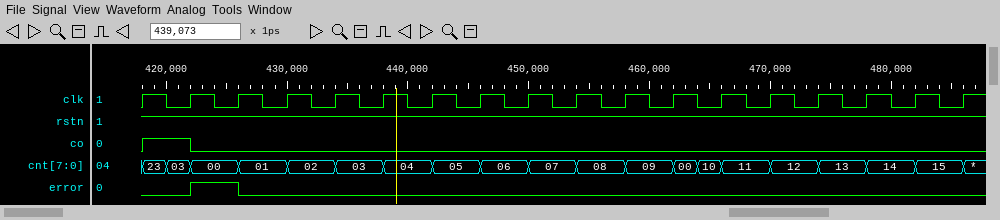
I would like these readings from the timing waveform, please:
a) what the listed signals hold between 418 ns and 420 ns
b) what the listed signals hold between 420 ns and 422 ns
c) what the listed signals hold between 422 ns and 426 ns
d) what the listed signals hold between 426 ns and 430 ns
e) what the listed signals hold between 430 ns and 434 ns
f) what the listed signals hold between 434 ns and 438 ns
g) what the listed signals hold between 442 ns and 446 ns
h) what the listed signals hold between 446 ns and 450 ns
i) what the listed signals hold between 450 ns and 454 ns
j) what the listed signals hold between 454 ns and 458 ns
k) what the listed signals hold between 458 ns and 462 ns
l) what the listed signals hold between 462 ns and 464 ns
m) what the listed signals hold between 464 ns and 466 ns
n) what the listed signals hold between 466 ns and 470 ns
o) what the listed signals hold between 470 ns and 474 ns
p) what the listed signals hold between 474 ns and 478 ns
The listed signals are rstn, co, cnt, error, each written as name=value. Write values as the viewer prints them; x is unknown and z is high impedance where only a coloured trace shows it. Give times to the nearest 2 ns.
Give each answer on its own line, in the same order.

rstn=1, co=1, cnt=23, error=0
rstn=1, co=1, cnt=03, error=0
rstn=1, co=0, cnt=00, error=1
rstn=1, co=0, cnt=01, error=0
rstn=1, co=0, cnt=02, error=0
rstn=1, co=0, cnt=03, error=0
rstn=1, co=0, cnt=05, error=0
rstn=1, co=0, cnt=06, error=0
rstn=1, co=0, cnt=07, error=0
rstn=1, co=0, cnt=08, error=0
rstn=1, co=0, cnt=09, error=0
rstn=1, co=0, cnt=00, error=0
rstn=1, co=0, cnt=10, error=0
rstn=1, co=0, cnt=11, error=0
rstn=1, co=0, cnt=12, error=0
rstn=1, co=0, cnt=13, error=0
